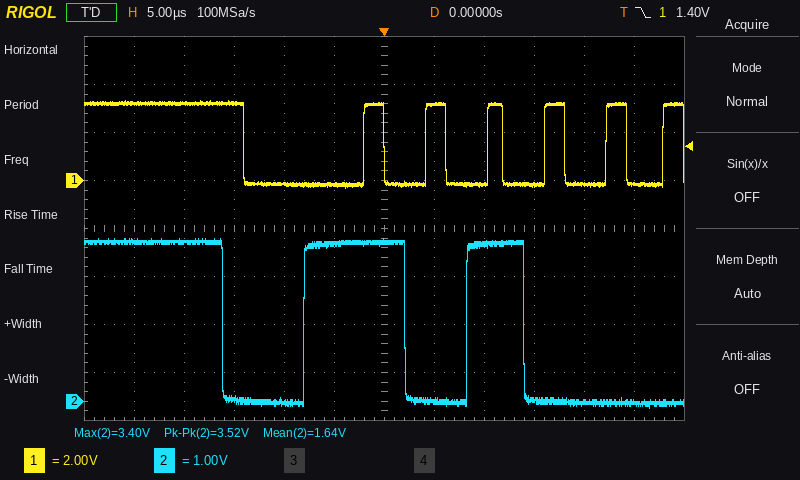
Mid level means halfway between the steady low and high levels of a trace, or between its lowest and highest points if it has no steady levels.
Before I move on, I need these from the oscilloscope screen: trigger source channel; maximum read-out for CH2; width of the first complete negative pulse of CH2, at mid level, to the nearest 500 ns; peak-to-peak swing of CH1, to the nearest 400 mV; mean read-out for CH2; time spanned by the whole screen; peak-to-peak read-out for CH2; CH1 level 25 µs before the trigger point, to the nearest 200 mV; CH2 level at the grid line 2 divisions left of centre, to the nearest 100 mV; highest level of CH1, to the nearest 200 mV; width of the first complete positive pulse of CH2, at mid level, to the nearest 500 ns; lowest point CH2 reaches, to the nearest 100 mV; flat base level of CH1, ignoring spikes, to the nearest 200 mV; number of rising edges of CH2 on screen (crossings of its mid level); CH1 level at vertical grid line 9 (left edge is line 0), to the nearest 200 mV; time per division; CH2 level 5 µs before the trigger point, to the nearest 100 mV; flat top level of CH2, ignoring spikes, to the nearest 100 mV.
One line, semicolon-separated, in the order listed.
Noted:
CH1; 3.40 V; 8.0 µs; 3.6 V; 1.64 V; 60 µs; 3.52 V; 3.2 V; 0.0 V; 3.4 V; 10.0 µs; -100 mV; -200 mV; 2; -200 mV; 5 µs; 3.3 V; 3.3 V
